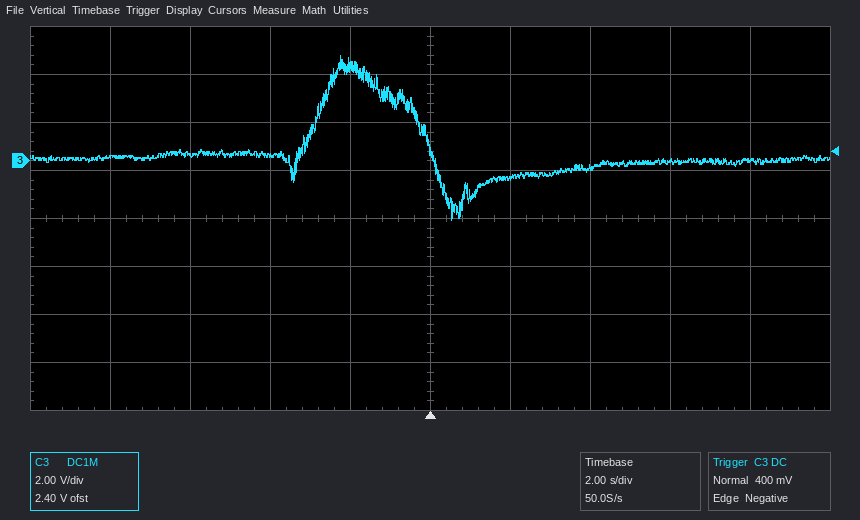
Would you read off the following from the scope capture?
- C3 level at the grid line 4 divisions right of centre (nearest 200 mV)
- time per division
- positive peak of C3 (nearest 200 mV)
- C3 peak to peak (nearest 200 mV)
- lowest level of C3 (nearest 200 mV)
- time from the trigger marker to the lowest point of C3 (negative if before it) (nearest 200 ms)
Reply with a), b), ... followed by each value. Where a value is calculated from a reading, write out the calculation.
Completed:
a) 0.0 V
b) 2 s
c) 4.4 V
d) 4.4 V − (-2.4 V) = 6.8 V
e) -2.4 V
f) +600 ms
